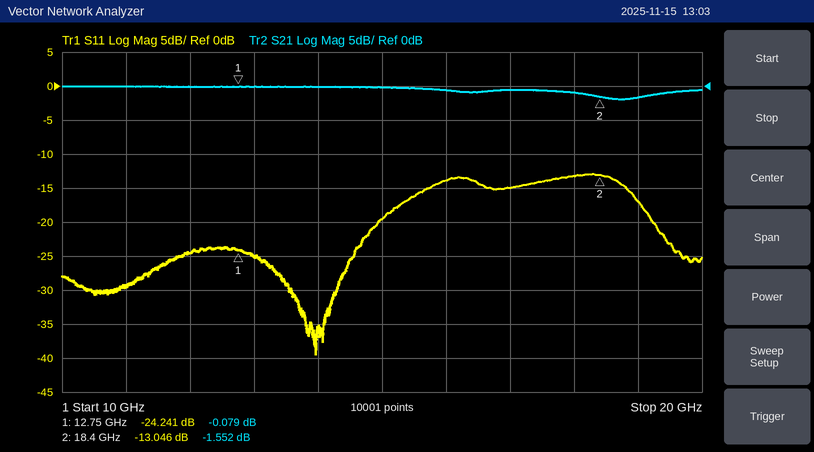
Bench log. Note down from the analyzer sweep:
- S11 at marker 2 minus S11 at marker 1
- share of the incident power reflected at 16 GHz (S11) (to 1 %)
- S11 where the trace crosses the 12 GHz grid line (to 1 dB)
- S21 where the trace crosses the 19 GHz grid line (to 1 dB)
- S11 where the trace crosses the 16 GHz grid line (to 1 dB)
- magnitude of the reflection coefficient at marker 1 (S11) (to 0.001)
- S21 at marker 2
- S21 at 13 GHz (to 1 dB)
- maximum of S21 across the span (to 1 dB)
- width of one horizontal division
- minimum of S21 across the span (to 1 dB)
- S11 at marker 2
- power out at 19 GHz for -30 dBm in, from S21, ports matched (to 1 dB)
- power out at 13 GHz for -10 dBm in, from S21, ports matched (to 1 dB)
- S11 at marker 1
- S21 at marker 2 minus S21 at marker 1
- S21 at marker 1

11.195 dB
4 %
-25 dB
-2 dB
-14 dB
0.061
-1.552 dB
0 dB
0 dB
1 GHz
-2 dB
-13.046 dB
-32 dBm
-10 dBm
-24.241 dB
-1.473 dB
-0.079 dB
